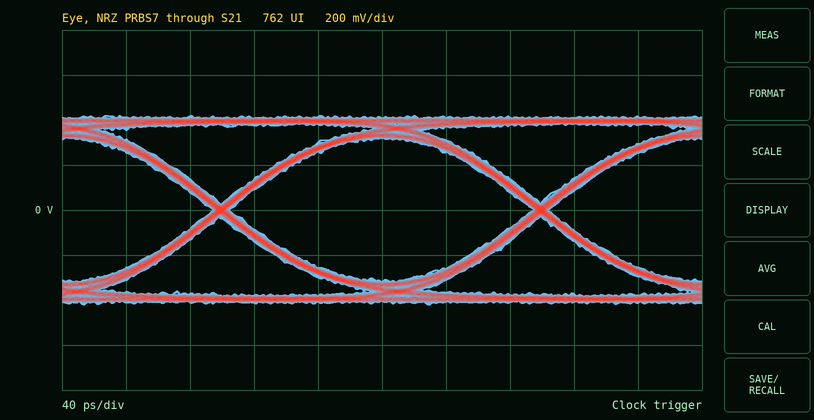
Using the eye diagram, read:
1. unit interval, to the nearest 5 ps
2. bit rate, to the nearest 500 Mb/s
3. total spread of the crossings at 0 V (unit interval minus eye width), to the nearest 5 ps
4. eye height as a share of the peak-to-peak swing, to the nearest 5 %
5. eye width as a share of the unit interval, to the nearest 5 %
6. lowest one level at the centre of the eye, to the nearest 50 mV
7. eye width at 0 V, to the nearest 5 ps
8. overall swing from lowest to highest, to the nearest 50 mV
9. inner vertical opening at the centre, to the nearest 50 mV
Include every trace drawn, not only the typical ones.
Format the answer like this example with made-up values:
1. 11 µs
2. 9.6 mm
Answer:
1. 200 ps
2. 5.0 Gb/s
3. 10 ps
4. 75 %
5. 95 %
6. 300 mV
7. 190 ps
8. 850 mV
9. 650 mV
